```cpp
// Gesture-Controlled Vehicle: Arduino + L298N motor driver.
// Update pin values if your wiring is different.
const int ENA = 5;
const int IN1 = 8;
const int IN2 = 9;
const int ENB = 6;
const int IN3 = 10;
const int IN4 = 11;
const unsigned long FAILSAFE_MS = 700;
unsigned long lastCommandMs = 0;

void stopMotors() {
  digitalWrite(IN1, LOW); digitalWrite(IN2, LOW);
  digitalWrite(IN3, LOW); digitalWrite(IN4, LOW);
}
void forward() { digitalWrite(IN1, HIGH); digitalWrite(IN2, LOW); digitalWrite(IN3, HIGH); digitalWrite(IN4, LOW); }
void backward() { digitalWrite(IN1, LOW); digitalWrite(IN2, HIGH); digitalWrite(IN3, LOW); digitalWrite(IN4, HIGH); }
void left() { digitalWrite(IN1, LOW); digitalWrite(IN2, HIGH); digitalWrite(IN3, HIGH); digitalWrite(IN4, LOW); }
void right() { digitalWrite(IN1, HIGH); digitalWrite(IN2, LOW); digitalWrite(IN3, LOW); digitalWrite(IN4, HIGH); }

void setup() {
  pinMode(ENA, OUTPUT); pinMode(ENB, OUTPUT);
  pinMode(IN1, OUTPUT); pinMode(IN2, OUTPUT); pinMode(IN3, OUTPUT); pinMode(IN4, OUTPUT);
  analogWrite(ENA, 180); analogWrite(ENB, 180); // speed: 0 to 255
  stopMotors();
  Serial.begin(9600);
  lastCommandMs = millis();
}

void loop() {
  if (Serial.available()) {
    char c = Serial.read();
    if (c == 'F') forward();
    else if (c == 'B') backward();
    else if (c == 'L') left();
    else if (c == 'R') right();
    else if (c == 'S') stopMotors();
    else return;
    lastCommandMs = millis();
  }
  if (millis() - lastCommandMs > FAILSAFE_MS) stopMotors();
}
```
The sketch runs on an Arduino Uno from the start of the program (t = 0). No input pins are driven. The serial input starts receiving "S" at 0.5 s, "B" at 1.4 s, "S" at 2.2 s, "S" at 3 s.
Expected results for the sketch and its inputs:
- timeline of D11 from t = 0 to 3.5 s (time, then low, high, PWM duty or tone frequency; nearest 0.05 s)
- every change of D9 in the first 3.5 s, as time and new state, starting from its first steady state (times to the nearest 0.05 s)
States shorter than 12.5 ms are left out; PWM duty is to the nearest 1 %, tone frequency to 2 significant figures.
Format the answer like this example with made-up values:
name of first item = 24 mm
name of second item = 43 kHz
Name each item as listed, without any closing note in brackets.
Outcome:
timeline of D11 from t = 0 to 3.5 s = 0 s low; 1.4 s high; 2.1 s low
every change of D9 in the first 3.5 s, as time and new state, starting from its first steady state = 0 s low; 1.4 s high; 2.1 s low
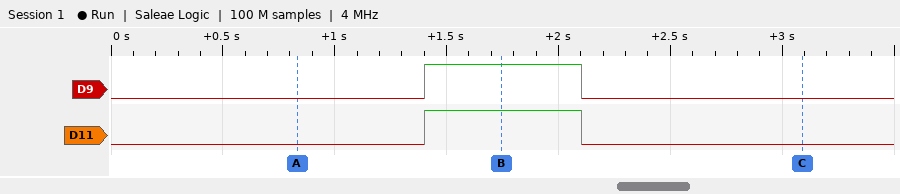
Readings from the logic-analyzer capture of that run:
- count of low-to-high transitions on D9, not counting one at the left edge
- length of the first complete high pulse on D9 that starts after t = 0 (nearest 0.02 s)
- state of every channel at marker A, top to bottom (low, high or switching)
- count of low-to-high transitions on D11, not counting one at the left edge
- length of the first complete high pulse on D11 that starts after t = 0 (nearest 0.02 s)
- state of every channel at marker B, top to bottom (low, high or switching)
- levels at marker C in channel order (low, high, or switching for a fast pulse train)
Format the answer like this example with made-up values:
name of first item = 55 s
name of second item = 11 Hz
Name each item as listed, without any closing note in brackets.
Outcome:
count of low-to-high transitions on D9, not counting one at the left edge = 1
length of the first complete high pulse on D9 that starts after t = 0 = 0.70 s
state of every channel at marker A, top to bottom = D9 low, D11 low
count of low-to-high transitions on D11, not counting one at the left edge = 1
length of the first complete high pulse on D11 that starts after t = 0 = 0.70 s
state of every channel at marker B, top to bottom = D9 high, D11 high
levels at marker C in channel order = D9 low, D11 low
